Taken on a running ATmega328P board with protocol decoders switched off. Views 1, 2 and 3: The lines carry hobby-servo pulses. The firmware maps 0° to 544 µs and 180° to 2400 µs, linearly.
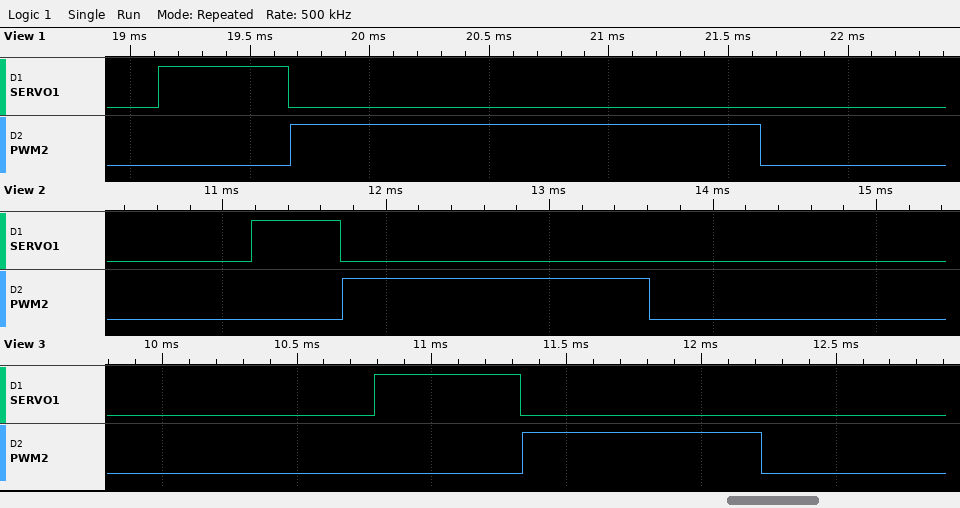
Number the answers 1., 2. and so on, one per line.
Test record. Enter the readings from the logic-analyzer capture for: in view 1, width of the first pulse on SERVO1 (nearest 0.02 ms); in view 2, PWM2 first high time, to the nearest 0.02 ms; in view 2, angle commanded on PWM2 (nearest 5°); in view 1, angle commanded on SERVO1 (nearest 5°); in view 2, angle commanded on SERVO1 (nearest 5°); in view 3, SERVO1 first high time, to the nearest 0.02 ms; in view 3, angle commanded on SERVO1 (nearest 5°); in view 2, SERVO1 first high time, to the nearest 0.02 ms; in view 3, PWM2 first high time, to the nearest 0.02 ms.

1. 0.54 ms
2. 1.88 ms
3. 130°
4. 0°
5. 0°
6. 0.54 ms
7. 0°
8. 0.54 ms
9. 0.88 ms
